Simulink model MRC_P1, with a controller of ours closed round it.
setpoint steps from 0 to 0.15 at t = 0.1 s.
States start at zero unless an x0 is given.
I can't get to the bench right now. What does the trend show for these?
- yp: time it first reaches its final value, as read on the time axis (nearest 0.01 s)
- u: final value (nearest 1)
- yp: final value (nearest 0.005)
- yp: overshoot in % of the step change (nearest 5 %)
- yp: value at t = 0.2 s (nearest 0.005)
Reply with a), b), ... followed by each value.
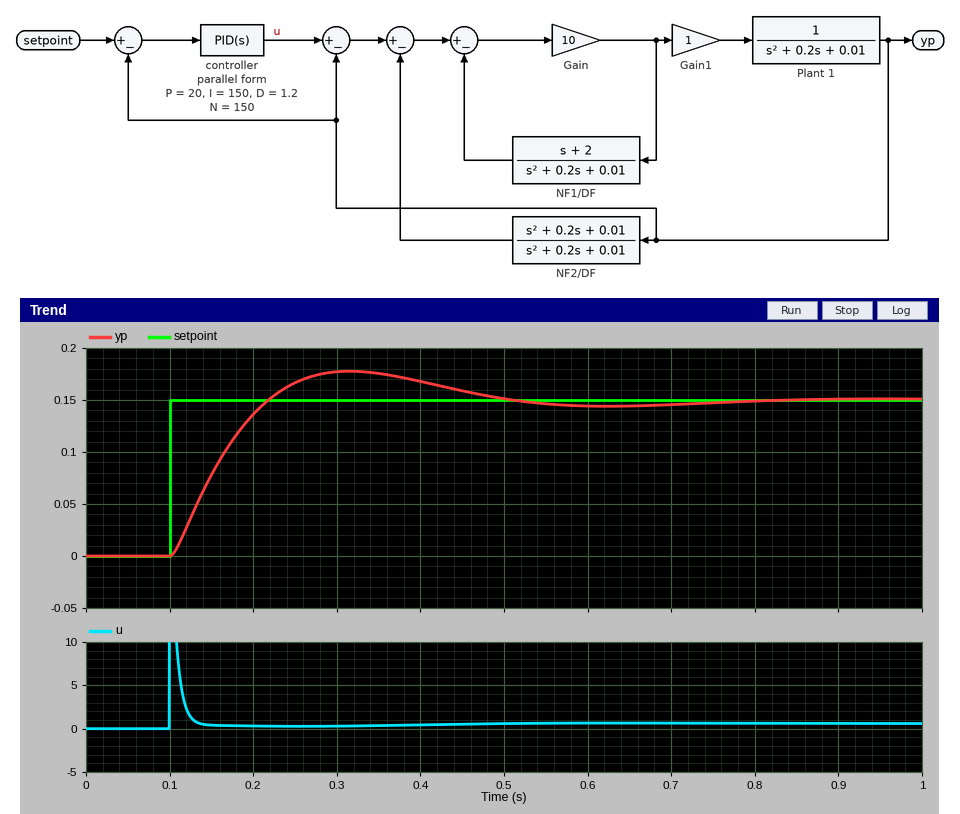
a) 0.22 s
b) 1
c) 0.150
d) 20 %
e) 0.135
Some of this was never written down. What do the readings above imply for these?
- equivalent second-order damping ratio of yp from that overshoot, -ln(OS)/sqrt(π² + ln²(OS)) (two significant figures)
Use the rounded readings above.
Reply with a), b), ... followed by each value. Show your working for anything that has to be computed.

a) ln(0.2) = -1.609; 1.609 / sqrt(9.870 + 2.590) = 0.46
